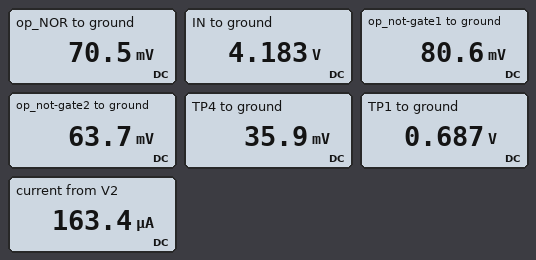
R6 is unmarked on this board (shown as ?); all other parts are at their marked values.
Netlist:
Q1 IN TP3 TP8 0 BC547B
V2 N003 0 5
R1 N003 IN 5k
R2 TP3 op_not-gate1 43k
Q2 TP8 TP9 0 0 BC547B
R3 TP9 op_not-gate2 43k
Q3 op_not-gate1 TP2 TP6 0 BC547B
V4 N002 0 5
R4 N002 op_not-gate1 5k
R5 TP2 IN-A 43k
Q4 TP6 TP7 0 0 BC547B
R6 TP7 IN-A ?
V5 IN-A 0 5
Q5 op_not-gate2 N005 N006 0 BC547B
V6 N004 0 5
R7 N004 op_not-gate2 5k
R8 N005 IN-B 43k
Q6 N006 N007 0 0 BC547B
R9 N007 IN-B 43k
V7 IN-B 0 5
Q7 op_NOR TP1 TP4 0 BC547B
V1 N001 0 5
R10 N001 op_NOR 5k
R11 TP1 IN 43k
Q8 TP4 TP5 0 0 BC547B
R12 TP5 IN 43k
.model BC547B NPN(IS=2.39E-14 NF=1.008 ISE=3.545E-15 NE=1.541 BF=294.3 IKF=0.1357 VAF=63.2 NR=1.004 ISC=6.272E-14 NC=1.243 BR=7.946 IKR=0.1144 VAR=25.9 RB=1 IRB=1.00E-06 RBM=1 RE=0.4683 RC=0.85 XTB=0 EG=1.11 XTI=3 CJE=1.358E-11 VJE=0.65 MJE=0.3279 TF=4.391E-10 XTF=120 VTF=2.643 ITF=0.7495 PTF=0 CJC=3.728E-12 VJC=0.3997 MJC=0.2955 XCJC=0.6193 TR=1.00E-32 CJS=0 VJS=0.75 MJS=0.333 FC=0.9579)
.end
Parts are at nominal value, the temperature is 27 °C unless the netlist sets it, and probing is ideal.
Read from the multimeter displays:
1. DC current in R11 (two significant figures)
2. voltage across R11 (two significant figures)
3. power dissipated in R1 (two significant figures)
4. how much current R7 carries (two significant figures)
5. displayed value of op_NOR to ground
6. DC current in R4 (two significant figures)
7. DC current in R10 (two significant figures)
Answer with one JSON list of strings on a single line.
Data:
["81 µA", "3.5 V", "130 µW", "990 µA", "70.5 mV", "980 µA", "990 µA"]
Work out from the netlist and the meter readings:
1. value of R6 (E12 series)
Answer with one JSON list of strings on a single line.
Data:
["100 kΩ"]
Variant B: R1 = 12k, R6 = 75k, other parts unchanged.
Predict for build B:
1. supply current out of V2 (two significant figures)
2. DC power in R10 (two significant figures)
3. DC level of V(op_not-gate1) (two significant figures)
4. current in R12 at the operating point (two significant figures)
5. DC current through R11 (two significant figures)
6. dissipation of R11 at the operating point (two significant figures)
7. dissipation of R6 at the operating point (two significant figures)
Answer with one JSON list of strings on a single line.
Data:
["130 µA", "4.8 mW", "74 mV", "65 µA", "64 µA", "180 µW", "250 µW"]
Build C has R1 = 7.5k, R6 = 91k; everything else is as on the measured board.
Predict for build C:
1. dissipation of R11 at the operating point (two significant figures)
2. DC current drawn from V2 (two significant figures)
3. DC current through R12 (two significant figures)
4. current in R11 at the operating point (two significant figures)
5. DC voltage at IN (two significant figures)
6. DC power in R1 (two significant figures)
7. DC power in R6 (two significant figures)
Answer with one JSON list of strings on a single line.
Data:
["240 µW", "150 µA", "75 µA", "74 µA", "3.9 V", "170 µW", "210 µW"]
